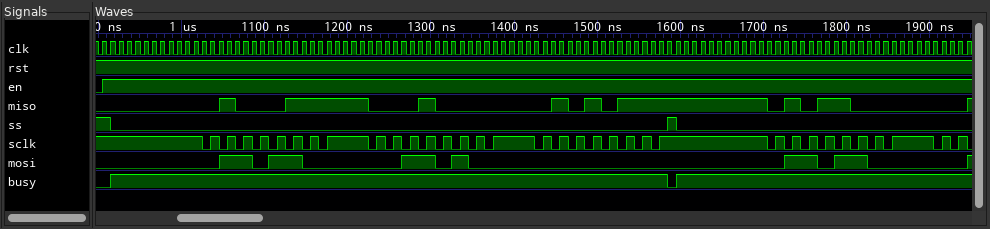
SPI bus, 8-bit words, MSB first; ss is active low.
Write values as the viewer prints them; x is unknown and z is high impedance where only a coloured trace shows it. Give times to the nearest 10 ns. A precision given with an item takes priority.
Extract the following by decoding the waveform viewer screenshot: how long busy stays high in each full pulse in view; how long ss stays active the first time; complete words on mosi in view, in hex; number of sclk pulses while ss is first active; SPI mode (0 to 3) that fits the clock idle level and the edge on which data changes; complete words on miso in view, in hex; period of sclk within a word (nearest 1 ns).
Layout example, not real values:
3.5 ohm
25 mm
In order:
670 ns
670 ns
6C, 34, 00, 6C
24
3
47, 10, 57, 58
20 ns
